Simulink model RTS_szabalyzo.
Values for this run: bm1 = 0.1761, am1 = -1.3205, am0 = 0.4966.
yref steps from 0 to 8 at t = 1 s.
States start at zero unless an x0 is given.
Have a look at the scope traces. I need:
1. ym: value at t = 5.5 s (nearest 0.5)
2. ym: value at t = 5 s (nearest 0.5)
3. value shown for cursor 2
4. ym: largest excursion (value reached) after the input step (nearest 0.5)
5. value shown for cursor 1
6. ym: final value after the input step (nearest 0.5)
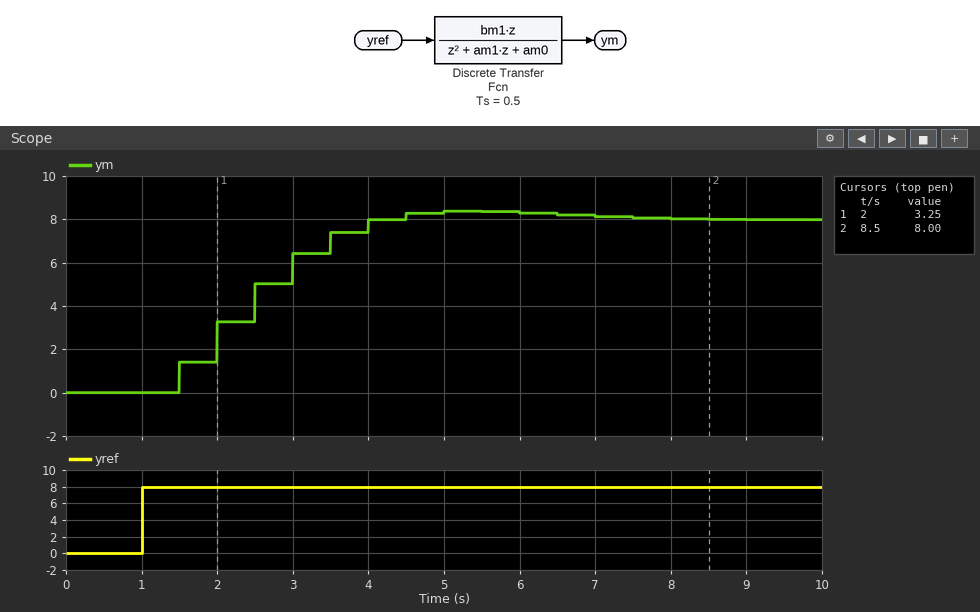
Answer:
8.5
8.5
8.00
8.5
3.25
8.0
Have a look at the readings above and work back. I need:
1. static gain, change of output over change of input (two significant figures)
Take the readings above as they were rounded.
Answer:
1.0
